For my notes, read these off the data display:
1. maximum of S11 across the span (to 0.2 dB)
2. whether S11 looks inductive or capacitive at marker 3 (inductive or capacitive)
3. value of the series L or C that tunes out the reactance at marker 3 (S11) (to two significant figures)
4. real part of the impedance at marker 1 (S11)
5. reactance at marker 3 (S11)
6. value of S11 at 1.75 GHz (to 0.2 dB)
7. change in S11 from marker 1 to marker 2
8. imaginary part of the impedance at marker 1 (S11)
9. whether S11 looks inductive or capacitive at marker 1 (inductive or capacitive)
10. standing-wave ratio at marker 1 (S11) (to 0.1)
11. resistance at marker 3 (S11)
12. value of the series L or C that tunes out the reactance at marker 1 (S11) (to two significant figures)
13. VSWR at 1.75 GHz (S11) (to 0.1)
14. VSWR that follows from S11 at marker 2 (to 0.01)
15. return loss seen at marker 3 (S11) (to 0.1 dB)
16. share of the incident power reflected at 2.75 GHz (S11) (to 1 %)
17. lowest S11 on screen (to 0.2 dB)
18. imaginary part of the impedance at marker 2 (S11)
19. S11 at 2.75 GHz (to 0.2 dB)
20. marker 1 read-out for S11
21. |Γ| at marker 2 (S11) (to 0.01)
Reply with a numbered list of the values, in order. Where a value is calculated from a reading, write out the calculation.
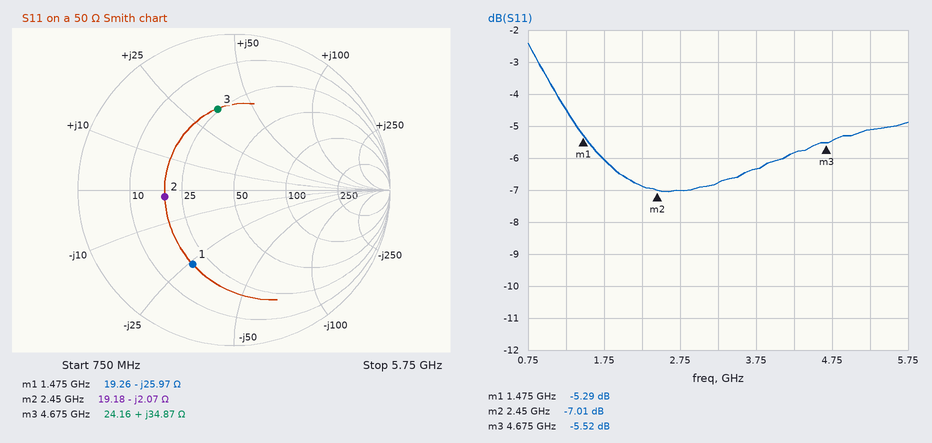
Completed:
1. -2.4 dB
2. inductive
3. C = 1/(2π × 4.675 GHz × 34.87 Ω) ≈ 976 fF, so 980 fF to two significant figures
4. 19.26 Ω
5. +34.87 Ω
6. -6.0 dB
7. -7.01 − (-5.29) = -1.72 dB
8. -25.97 Ω
9. capacitive
10. 3.4
11. 24.16 Ω
12. L = 25.97 Ω/(2π × 1.475 GHz) ≈ 2.8 nH
13. |Γ| = 10^(-6/20) = 0.5012; VSWR = (1 + 0.5012)/(1 − 0.5012) ≈ 3.0
14. (1 + 0.4462)/(1 − 0.4462) ≈ 2.61
15. 5.5 dB
16. 10^(-7/10) ≈ 20 %
17. -7.0 dB
18. -2.07 Ω
19. -7.0 dB
20. -5.29 dB
21. 0.45
